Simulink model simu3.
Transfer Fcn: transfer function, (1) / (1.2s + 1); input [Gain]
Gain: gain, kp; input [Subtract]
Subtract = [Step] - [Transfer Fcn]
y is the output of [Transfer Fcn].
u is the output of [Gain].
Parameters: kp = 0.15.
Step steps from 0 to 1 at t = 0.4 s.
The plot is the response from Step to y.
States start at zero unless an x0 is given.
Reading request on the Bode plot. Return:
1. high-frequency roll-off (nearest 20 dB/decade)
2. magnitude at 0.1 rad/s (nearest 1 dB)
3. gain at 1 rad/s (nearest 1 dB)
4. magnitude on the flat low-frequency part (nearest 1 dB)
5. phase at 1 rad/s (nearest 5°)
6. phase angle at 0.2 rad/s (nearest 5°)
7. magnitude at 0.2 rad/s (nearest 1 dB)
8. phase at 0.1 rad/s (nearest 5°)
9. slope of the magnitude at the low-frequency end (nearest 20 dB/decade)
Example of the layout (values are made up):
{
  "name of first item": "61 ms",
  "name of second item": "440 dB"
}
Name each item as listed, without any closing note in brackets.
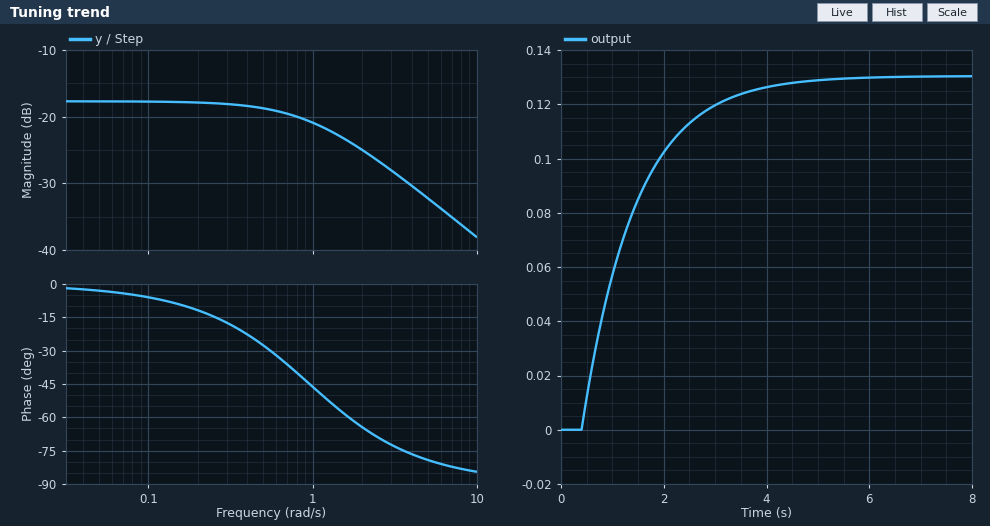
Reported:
{
  "high-frequency roll-off": "-20 dB/decade",
  "magnitude at 0.1 rad/s": "-18 dB",
  "gain at 1 rad/s": "-21 dB",
  "magnitude on the flat low-frequency part": "-18 dB",
  "phase at 1 rad/s": "-45°",
  "phase angle at 0.2 rad/s": "-10°",
  "magnitude at 0.2 rad/s": "-18 dB",
  "phase at 0.1 rad/s": "-5°",
  "slope of the magnitude at the low-frequency end": "0 dB/decade"
}
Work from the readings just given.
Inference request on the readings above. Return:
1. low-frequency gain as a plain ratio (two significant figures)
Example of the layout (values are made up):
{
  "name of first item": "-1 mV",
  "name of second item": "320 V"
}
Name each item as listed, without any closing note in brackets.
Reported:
{
  "low-frequency gain as a plain ratio": "0.13"
}
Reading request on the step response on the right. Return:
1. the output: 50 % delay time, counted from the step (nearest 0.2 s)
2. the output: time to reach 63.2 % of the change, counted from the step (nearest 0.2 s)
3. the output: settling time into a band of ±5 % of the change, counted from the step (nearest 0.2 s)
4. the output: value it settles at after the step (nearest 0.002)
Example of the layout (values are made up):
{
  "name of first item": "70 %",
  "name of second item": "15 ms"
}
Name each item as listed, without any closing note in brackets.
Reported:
{
  "the output: 50 % delay time, counted from the step": "0.8 s",
  "the output: time to reach 63.2 % of the change, counted from the step": "1.0 s",
  "the output: settling time into a band of ±5 % of the change, counted from the step": "3.2 s",
  "the output: value it settles at after the step": "0.130"
}
